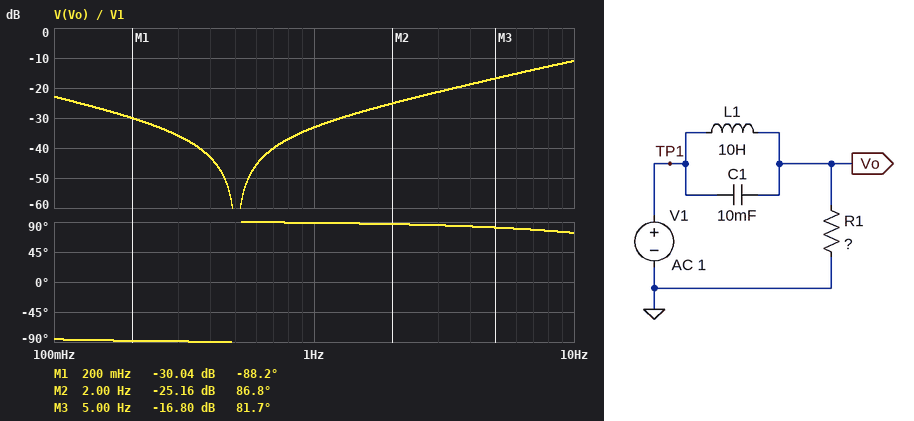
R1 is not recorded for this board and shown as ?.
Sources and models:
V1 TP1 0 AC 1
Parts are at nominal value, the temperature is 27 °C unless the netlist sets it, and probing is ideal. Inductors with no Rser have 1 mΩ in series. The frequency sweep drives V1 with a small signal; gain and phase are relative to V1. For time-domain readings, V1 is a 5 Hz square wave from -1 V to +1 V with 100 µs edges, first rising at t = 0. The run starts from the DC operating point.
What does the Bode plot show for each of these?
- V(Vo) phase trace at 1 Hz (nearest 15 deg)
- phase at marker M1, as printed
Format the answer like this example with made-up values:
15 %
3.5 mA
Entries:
90 deg
-88.2 deg
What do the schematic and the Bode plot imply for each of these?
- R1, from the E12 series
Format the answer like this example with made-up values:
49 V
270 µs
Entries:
0.47 Ω
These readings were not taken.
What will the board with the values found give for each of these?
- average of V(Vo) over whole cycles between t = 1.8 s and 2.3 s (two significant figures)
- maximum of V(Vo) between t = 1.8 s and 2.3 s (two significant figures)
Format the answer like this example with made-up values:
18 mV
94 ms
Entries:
-910 mV
1.1 V
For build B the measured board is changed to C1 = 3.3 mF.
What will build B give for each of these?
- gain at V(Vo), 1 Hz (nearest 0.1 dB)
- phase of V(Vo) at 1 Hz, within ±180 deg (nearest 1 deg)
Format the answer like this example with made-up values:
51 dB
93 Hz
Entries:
-52.9 dB
90 deg
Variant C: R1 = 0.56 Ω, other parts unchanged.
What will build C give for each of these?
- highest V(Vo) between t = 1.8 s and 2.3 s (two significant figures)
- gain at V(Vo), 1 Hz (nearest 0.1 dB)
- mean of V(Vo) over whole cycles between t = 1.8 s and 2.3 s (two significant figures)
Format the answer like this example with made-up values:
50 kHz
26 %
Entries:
1.1 V
-31.6 dB
-890 mV
